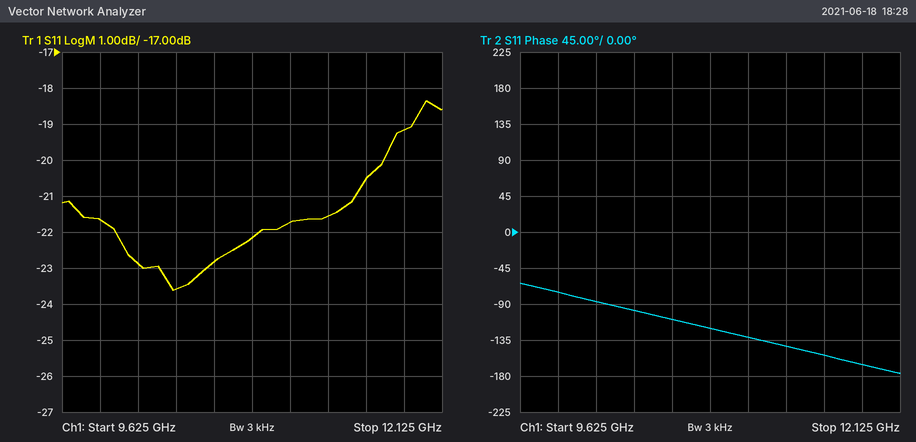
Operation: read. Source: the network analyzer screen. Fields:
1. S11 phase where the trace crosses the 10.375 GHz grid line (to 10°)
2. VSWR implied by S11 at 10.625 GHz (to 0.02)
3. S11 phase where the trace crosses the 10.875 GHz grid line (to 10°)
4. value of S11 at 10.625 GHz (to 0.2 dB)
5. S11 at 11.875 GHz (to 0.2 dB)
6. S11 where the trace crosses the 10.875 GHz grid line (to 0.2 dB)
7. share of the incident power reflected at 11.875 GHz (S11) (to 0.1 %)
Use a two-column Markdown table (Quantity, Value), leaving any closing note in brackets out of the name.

| Quantity | Value |
|---|---|
| S11 phase where the trace crosses the 10.375 GHz grid line | -100° |
| VSWR implied by S11 at 10.625 GHz | 1.16 |
| S11 phase where the trace crosses the 10.875 GHz grid line | -120° |
| value of S11 at 10.625 GHz | -22.8 dB |
| S11 at 11.875 GHz | -19.2 dB |
| S11 where the trace crosses the 10.875 GHz grid line | -22.2 dB |
| share of the incident power reflected at 11.875 GHz (S11) | 1.2 % |
